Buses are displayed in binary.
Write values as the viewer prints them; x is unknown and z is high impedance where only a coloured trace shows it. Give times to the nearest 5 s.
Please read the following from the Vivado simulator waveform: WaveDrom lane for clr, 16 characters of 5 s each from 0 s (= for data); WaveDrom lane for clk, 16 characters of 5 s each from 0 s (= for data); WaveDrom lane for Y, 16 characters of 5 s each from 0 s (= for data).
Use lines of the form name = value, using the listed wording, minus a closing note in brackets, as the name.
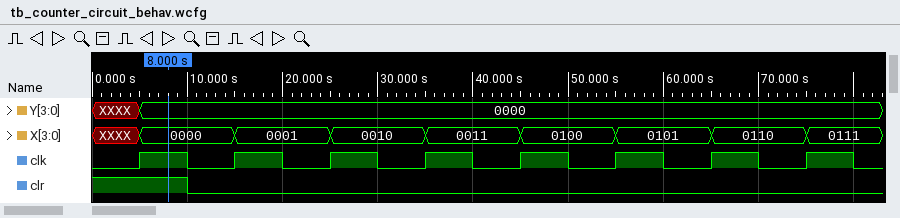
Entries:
WaveDrom lane for clr, 16 characters of 5 s each from 0 s = {name: 'clr', wave: '1.0.............'}
WaveDrom lane for clk, 16 characters of 5 s each from 0 s = {name: 'clk', wave: '0101010101010101'}
WaveDrom lane for Y, 16 characters of 5 s each from 0 s = {name: 'Y', wave: 'x=..............', data: '0000'}
